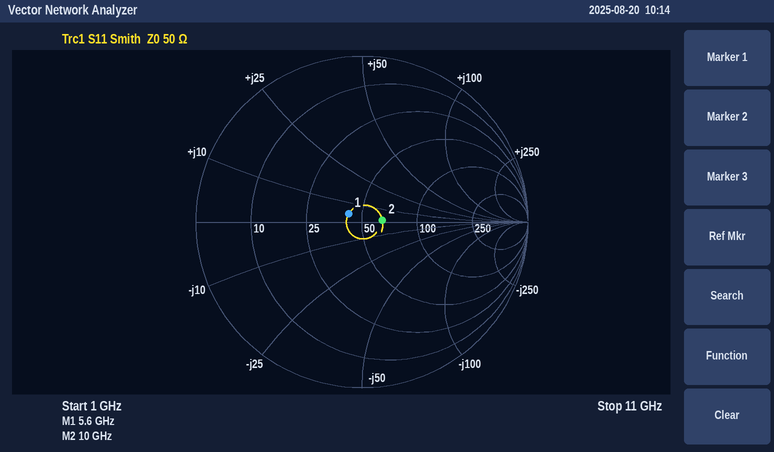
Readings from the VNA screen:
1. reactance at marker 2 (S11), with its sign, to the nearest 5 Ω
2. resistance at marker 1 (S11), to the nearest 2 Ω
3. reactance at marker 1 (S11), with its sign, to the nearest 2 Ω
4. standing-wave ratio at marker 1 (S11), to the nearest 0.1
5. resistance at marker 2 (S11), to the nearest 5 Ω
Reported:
0 Ω
42 Ω
+4 Ω
1.2
65 Ω
